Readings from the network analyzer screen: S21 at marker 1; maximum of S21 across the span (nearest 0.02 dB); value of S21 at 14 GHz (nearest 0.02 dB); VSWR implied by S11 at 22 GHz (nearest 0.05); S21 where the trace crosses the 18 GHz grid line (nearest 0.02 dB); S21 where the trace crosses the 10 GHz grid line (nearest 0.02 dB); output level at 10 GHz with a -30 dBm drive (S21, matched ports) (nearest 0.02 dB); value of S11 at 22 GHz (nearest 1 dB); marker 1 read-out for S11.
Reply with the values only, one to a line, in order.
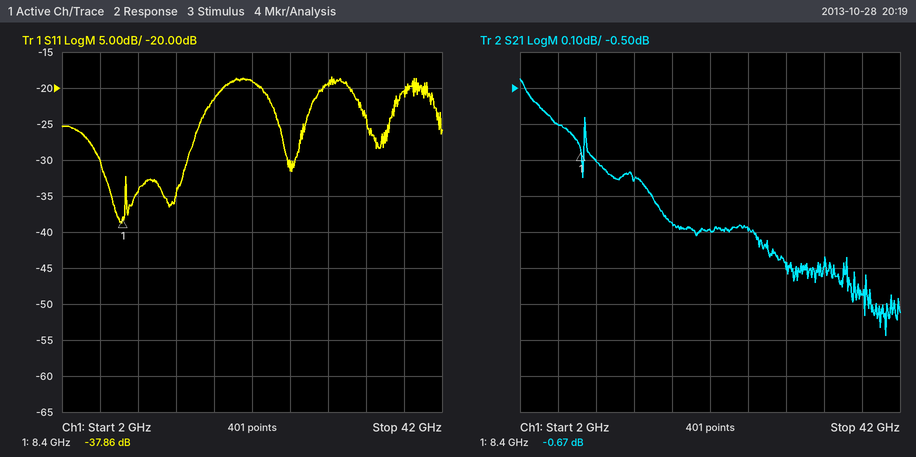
-0.67 dB
-0.48 dB
-0.76 dB
1.25
-0.88 dB
-0.70 dB
-30.70 dBm
-19 dB
-37.86 dB
